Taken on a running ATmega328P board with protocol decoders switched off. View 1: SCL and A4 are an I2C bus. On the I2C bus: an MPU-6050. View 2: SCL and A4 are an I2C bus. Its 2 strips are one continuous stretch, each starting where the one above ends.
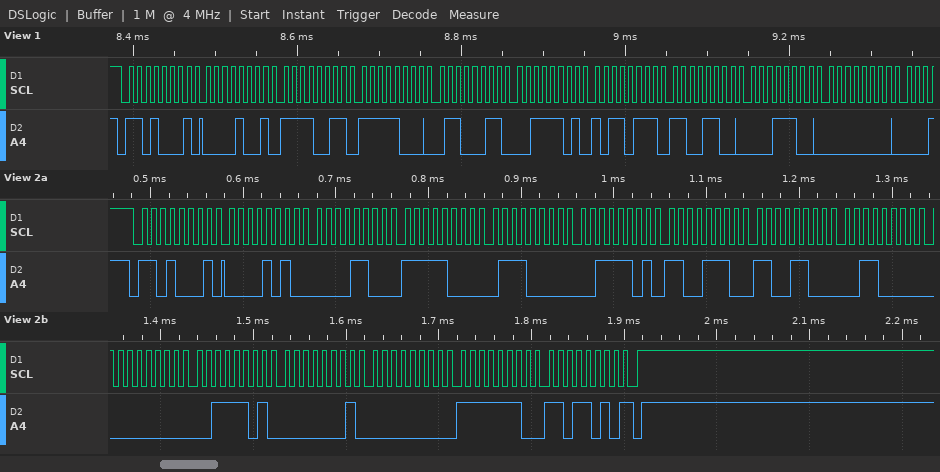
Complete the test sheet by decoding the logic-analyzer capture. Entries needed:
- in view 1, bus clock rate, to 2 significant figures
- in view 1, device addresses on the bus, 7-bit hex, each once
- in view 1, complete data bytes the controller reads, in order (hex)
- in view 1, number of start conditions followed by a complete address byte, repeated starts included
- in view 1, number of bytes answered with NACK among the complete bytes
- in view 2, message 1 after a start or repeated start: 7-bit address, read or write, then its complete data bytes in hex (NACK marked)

100 kHz
0x68
09 F3 F8 63 3D B7 CC 1C 00
1
0
0x68 read: 0A 0C F8 70 3D CE CC 30 00 3D 01 00 FE DA NACK
